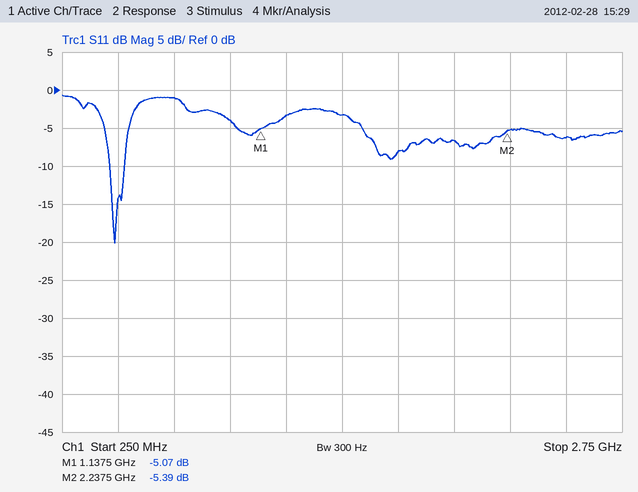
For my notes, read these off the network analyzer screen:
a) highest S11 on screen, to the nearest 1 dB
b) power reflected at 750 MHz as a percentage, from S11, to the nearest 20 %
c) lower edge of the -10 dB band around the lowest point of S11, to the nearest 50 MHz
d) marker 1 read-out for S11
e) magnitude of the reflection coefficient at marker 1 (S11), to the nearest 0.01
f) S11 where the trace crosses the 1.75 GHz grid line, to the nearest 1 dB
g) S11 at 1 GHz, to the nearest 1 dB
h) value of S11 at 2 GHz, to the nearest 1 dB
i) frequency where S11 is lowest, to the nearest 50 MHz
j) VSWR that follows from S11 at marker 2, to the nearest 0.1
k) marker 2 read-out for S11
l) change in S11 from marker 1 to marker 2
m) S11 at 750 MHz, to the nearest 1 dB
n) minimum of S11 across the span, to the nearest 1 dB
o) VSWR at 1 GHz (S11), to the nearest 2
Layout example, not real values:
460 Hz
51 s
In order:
-1 dB
80 %
450 MHz
-5.07 dB
0.56
-8 dB
-4 dB
-7 dB
500 MHz
3.3
-5.39 dB
-0.32 dB
-1 dB
-20 dB
4
